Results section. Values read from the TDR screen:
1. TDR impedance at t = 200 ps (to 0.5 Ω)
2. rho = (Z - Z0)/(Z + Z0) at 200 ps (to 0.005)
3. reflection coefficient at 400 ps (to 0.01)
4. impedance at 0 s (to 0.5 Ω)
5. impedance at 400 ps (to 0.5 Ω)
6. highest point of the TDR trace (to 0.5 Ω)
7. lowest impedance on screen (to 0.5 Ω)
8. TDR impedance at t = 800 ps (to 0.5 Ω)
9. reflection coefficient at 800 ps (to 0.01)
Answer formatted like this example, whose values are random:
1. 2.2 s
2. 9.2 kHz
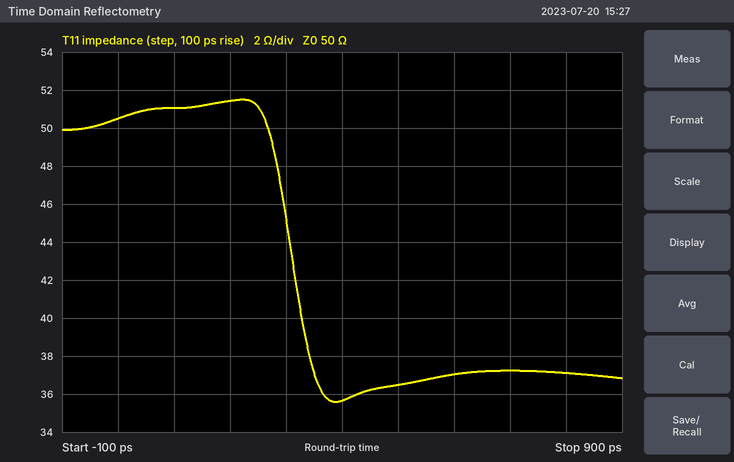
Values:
1. 51.5 Ω
2. +0.015
3. -0.17
4. 50.5 Ω
5. 35.5 Ω
6. 51.5 Ω
7. 35.5 Ω
8. 37.0 Ω
9. -0.15
